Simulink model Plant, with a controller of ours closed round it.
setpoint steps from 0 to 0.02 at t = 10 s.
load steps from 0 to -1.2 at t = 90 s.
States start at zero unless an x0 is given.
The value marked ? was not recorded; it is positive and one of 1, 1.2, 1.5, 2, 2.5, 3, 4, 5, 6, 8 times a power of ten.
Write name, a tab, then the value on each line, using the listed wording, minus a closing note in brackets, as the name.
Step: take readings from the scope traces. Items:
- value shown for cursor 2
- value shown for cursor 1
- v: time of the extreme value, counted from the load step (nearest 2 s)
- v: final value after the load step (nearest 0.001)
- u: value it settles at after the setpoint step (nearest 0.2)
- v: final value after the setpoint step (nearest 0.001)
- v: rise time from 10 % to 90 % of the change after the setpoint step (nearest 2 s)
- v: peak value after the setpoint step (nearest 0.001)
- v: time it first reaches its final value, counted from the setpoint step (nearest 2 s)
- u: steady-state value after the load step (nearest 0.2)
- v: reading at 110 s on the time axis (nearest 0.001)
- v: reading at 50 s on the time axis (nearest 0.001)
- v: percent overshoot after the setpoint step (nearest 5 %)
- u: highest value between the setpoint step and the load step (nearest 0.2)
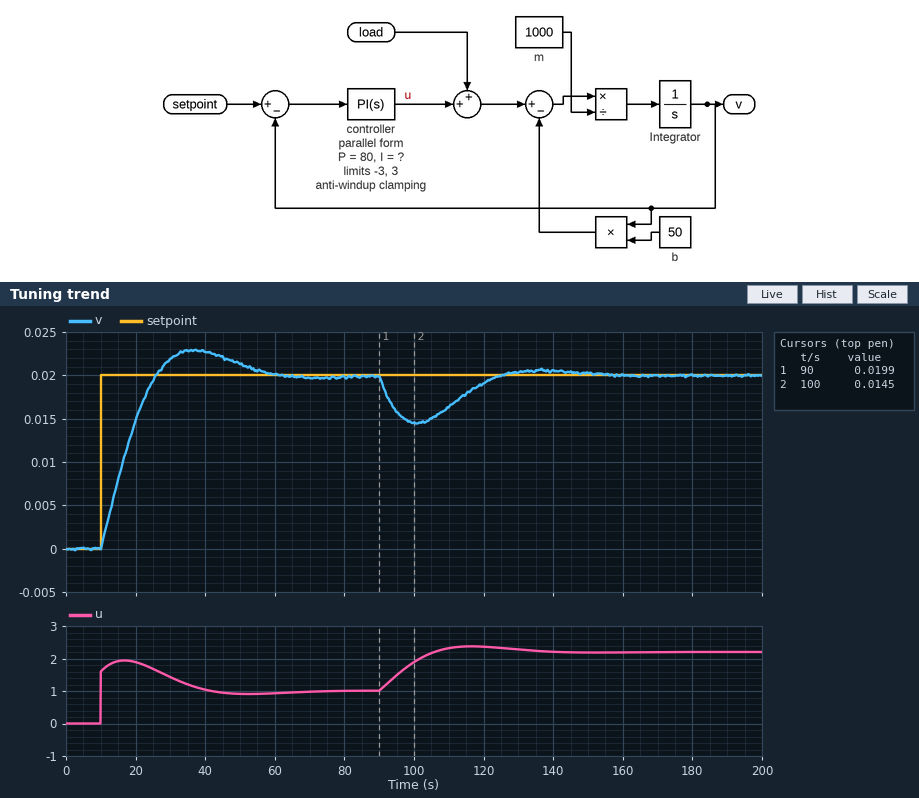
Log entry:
value shown for cursor 2	0.0145
value shown for cursor 1	0.0199
v: time of the extreme value, counted from the load step	10 s
v: final value after the load step	0.020
u: value it settles at after the setpoint step	1.0
v: final value after the setpoint step	0.020
v: rise time from 10 % to 90 % of the change after the setpoint step	12 s
v: peak value after the setpoint step	0.023
v: time it first reaches its final value, counted from the setpoint step	16 s
u: steady-state value after the load step	2.2
v: reading at 110 s on the time axis	0.016
v: reading at 50 s on the time axis	0.021
v: percent overshoot after the setpoint step	15 %
u: highest value between the setpoint step and the load step	2.0
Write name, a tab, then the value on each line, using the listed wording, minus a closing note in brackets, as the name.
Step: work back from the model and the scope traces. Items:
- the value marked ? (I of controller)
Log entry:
the value marked ?	12
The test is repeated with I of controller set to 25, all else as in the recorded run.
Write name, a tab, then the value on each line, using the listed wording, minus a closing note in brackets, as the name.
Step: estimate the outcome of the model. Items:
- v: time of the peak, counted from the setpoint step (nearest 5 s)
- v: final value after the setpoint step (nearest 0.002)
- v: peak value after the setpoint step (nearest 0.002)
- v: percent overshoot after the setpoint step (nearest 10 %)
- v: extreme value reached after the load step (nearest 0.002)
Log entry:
v: time of the peak, counted from the setpoint step	20 s
v: final value after the setpoint step	0.020
v: peak value after the setpoint step	0.026
v: percent overshoot after the setpoint step	30 %
v: extreme value reached after the load step	0.016
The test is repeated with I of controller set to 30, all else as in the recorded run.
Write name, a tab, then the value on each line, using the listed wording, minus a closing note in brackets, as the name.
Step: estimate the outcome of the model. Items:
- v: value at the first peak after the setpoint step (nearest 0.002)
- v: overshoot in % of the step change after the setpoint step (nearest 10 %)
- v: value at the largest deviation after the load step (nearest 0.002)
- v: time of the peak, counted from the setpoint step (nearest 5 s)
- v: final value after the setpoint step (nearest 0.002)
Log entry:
v: value at the first peak after the setpoint step	0.026
v: overshoot in % of the step change after the setpoint step	30 %
v: value at the largest deviation after the load step	0.016
v: time of the peak, counted from the setpoint step	15 s
v: final value after the setpoint step	0.020
